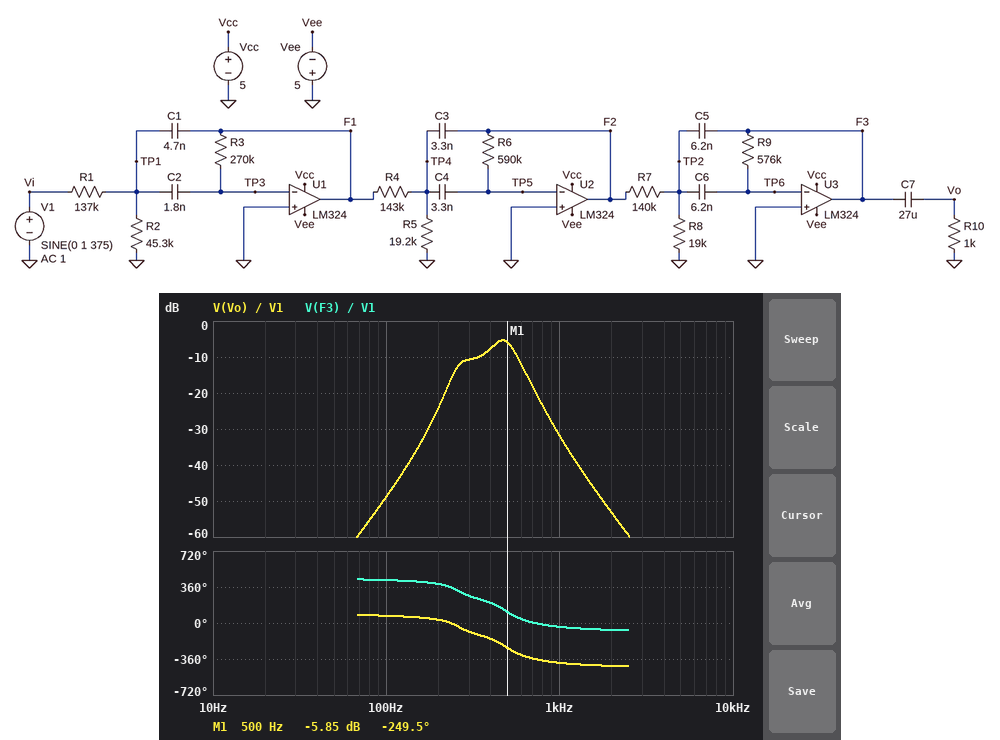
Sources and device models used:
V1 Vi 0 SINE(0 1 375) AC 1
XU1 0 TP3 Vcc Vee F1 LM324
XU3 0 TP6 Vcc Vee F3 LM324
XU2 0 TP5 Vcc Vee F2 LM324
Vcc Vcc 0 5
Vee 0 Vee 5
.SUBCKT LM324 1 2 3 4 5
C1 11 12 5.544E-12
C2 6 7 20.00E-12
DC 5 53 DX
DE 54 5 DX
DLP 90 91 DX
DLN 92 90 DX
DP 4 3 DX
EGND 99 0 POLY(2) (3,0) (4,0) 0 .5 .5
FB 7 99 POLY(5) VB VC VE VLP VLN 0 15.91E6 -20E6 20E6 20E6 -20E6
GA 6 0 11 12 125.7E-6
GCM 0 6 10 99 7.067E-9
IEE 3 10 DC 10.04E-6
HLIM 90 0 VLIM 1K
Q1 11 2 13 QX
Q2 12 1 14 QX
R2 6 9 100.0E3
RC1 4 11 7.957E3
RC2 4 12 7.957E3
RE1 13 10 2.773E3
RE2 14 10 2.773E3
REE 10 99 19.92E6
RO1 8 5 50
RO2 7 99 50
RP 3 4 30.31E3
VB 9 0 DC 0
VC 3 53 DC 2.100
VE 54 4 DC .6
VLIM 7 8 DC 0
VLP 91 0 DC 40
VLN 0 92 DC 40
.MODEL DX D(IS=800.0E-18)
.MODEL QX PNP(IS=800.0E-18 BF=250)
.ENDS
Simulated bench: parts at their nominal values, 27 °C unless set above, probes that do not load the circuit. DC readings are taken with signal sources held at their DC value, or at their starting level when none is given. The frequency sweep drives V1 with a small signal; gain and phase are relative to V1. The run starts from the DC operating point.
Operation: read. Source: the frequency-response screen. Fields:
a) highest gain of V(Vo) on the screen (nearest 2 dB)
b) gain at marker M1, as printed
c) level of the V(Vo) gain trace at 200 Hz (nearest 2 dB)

-6 dB
-5.85 dB
-24 dB
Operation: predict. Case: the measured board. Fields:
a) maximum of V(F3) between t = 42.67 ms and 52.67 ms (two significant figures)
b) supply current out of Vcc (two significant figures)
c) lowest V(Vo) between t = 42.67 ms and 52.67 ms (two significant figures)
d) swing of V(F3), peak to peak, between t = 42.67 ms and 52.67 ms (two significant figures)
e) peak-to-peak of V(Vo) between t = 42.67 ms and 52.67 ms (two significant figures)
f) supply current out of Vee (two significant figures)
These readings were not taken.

350 mV
1.0 mA
-360 mV
730 mV
730 mV
1.0 mA
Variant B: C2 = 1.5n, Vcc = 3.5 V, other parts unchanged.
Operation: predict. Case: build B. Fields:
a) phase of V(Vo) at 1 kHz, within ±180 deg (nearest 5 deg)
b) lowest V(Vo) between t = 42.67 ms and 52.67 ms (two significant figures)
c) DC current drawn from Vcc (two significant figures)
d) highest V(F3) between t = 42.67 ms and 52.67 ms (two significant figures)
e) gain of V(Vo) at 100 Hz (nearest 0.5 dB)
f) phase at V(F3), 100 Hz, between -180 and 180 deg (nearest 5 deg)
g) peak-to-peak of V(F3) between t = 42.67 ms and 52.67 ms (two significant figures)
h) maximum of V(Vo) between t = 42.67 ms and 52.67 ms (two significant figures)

-30 deg
-290 mV
870 µA
280 mV
-50.5 dB
70 deg
580 mV
290 mV
